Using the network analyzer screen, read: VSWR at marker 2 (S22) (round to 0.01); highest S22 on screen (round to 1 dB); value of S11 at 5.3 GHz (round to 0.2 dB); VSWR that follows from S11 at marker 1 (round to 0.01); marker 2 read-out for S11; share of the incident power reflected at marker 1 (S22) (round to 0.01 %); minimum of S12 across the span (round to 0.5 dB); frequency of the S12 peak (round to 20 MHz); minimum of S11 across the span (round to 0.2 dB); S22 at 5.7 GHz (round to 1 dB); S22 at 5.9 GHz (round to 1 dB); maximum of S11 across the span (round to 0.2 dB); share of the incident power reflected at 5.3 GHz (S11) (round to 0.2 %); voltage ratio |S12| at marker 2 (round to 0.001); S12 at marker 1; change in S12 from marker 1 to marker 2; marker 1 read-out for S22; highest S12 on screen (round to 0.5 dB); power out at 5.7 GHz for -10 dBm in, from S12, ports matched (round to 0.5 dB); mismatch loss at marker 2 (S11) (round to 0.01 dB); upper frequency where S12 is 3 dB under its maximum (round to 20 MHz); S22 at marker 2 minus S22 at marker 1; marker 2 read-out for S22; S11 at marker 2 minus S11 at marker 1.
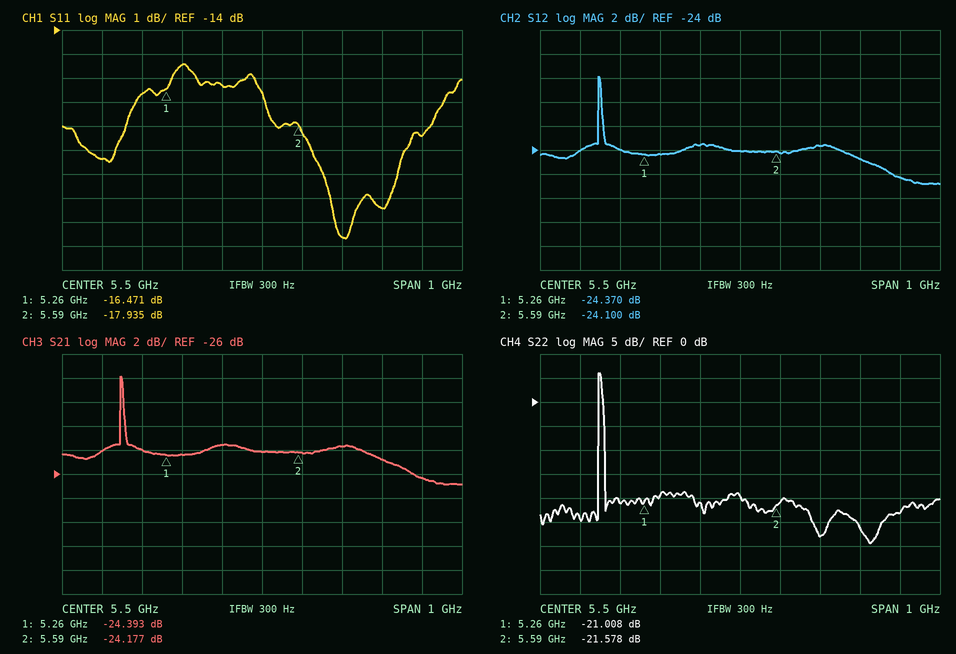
1.18
6 dB
-15.4 dB
1.35
-17.935 dB
0.79 %
-27.0 dB
5.14 GHz
-22.6 dB
-28 dB
-23 dB
-15.4 dB
2.8 %
0.062
-24.370 dB
0.270 dB
-21.008 dB
-18.0 dB
-33.5 dBm
0.07 dB
5.16 GHz
-0.570 dB
-21.578 dB
-1.464 dB
